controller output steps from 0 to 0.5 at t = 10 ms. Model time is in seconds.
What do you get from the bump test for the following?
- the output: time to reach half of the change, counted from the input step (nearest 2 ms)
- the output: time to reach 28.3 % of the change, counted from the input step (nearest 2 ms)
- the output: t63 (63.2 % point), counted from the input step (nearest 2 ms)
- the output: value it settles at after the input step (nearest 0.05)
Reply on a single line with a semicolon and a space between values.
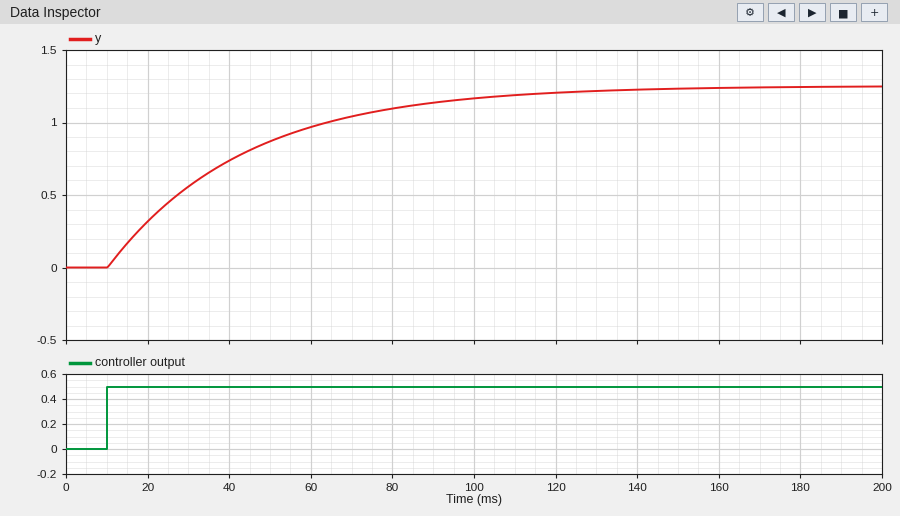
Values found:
24 ms; 12 ms; 34 ms; 1.25
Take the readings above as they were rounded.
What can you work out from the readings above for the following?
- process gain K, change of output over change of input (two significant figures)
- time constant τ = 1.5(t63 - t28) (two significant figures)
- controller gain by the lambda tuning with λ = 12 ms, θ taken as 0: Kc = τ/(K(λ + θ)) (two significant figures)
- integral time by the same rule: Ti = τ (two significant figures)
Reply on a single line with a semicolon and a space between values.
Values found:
2.5; 33 ms; 1.1; 33 ms
